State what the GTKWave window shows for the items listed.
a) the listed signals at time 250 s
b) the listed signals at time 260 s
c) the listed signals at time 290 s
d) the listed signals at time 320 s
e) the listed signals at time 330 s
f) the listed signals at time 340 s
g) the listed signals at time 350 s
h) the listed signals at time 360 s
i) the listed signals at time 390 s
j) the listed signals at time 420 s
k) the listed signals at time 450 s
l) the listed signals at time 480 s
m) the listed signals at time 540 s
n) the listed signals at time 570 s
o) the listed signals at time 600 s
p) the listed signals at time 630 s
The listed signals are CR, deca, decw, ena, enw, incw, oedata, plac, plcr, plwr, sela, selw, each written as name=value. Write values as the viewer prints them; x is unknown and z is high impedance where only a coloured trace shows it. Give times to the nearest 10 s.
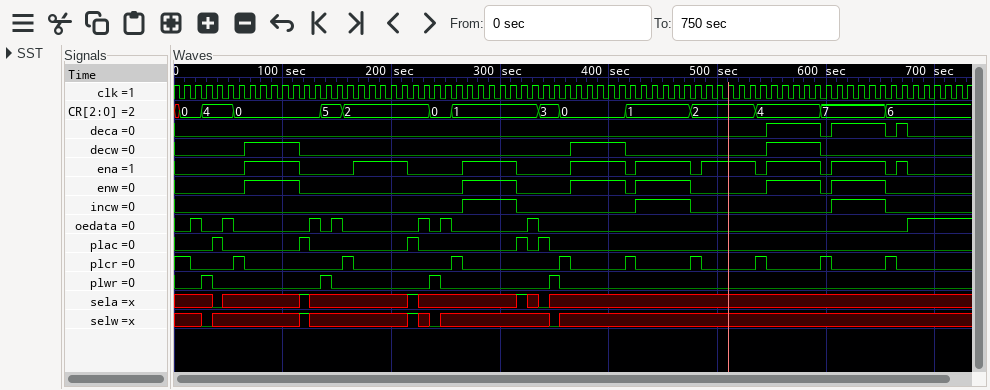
CR=0, deca=0, decw=0, ena=0, enw=0, incw=0, oedata=1, plac=0, plcr=0, plwr=0, sela=x, selw=x
CR=1, deca=0, decw=0, ena=0, enw=0, incw=0, oedata=0, plac=0, plcr=1, plwr=0, sela=x, selw=x
CR=1, deca=0, decw=0, ena=1, enw=1, incw=1, oedata=0, plac=0, plcr=0, plwr=0, sela=x, selw=x
CR=1, deca=0, decw=0, ena=0, enw=0, incw=0, oedata=0, plac=1, plcr=0, plwr=0, sela=1, selw=x
CR=1, deca=0, decw=0, ena=0, enw=0, incw=0, oedata=1, plac=0, plcr=0, plwr=0, sela=x, selw=x
CR=3, deca=0, decw=0, ena=0, enw=0, incw=0, oedata=0, plac=1, plcr=0, plwr=0, sela=0, selw=x
CR=3, deca=0, decw=0, ena=0, enw=0, incw=0, oedata=0, plac=0, plcr=0, plwr=1, sela=x, selw=0
CR=0, deca=0, decw=0, ena=0, enw=0, incw=0, oedata=0, plac=0, plcr=1, plwr=0, sela=x, selw=x
CR=0, deca=0, decw=1, ena=1, enw=1, incw=0, oedata=0, plac=0, plcr=0, plwr=0, sela=x, selw=x
CR=1, deca=0, decw=0, ena=0, enw=0, incw=0, oedata=0, plac=0, plcr=1, plwr=0, sela=x, selw=x
CR=1, deca=0, decw=0, ena=1, enw=1, incw=1, oedata=0, plac=0, plcr=0, plwr=0, sela=x, selw=x
CR=2, deca=0, decw=0, ena=0, enw=0, incw=0, oedata=0, plac=0, plcr=1, plwr=0, sela=x, selw=x
CR=4, deca=0, decw=0, ena=0, enw=0, incw=0, oedata=0, plac=0, plcr=1, plwr=0, sela=x, selw=x
CR=4, deca=1, decw=1, ena=1, enw=1, incw=0, oedata=0, plac=0, plcr=0, plwr=0, sela=x, selw=x
CR=7, deca=0, decw=0, ena=0, enw=0, incw=0, oedata=0, plac=0, plcr=1, plwr=0, sela=x, selw=x
CR=7, deca=1, decw=0, ena=1, enw=1, incw=1, oedata=0, plac=0, plcr=0, plwr=0, sela=x, selw=x
